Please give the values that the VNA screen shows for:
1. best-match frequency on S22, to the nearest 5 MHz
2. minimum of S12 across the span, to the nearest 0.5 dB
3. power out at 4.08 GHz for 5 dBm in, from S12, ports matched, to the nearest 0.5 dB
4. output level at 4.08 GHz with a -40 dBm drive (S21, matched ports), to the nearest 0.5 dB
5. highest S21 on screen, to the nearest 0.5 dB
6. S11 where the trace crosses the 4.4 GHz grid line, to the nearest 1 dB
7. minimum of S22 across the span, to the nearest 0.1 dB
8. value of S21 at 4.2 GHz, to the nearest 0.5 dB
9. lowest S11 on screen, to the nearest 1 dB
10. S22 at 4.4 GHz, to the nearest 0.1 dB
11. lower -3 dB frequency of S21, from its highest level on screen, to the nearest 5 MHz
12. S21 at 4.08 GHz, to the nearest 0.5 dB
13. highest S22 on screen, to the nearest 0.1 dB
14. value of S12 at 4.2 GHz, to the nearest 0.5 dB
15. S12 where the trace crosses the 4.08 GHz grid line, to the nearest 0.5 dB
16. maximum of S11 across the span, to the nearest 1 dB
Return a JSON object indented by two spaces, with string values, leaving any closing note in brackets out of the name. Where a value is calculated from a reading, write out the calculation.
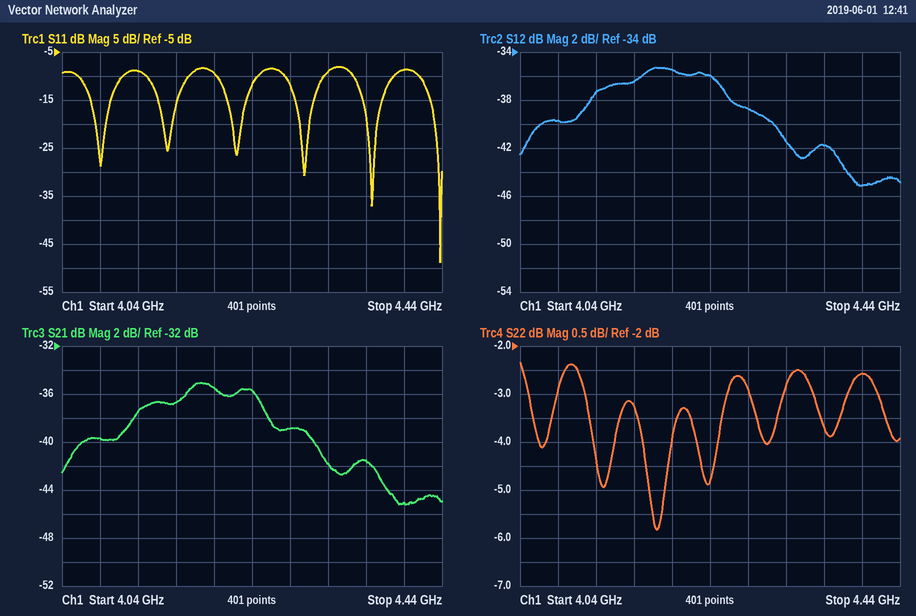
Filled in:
{
  "best-match frequency on S22, to the nearest 5 MHz": "4.185 GHz",
  "minimum of S12 across the span, to the nearest 0.5 dB": "-45.0 dB",
  "power out at 4.08 GHz for 5 dBm in, from S12, ports matched, to the nearest 0.5 dB": "5 dBm + (-39.5 dB) = -34.5 dBm",
  "output level at 4.08 GHz with a -40 dBm drive (S21, matched ports), to the nearest 0.5 dB": "-40 dBm + (-39.5 dB) = -79.5 dBm",
  "highest S21 on screen, to the nearest 0.5 dB": "-35.0 dB",
  "S11 where the trace crosses the 4.4 GHz grid line, to the nearest 1 dB": "-9 dB",
  "minimum of S22 across the span, to the nearest 0.1 dB": "-5.8 dB",
  "value of S21 at 4.2 GHz, to the nearest 0.5 dB": "-35.5 dB",
  "lowest S11 on screen, to the nearest 1 dB": "-49 dB",
  "S22 at 4.4 GHz, to the nearest 0.1 dB": "-2.6 dB",
  "lower -3 dB frequency of S21, from its highest level on screen, to the nearest 5 MHz": "4.115 GHz",
  "S21 at 4.08 GHz, to the nearest 0.5 dB": "-39.5 dB",
  "highest S22 on screen, to the nearest 0.1 dB": "-2.3 dB",
  "value of S12 at 4.2 GHz, to the nearest 0.5 dB": "-35.5 dB",
  "S12 where the trace crosses the 4.08 GHz grid line, to the nearest 0.5 dB": "-39.5 dB",
  "maximum of S11 across the span, to the nearest 1 dB": "-8 dB"
}
